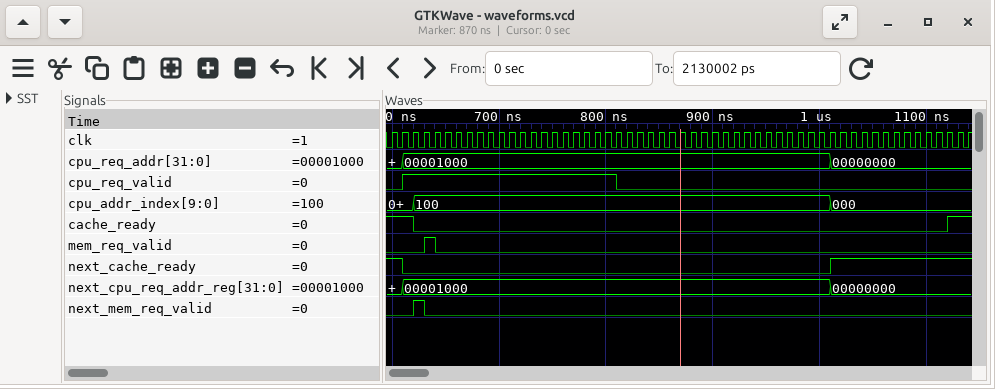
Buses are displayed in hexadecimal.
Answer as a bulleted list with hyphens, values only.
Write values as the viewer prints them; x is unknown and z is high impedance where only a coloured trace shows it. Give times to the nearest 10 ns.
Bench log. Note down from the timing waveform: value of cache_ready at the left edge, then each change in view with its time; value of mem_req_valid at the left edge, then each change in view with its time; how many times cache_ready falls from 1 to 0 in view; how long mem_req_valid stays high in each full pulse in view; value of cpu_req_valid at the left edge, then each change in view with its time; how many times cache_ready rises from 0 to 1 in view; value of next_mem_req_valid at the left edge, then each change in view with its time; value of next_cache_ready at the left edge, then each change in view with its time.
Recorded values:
- 1, 0 at 620 ns, 1 at 1120 ns
- 0, 1 at 630 ns, 0 at 640 ns
- 1
- 10 ns
- 0, 1 at 610 ns, 0 at 810 ns
- 1
- 0, 1 at 620 ns, 0 at 630 ns
- 1, 0 at 610 ns, 1 at 1010 ns
